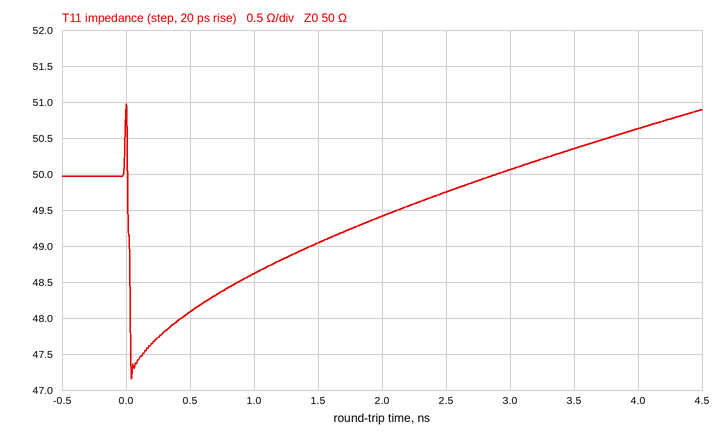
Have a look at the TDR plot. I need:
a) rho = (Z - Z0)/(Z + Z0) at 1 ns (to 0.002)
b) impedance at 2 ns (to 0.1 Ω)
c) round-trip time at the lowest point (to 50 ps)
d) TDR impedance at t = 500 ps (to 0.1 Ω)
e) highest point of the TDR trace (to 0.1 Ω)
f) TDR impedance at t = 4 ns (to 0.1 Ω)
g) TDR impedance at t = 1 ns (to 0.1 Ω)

-0.014
49.4 Ω
50 ps
48.1 Ω
51.0 Ω
50.6 Ω
48.6 Ω
